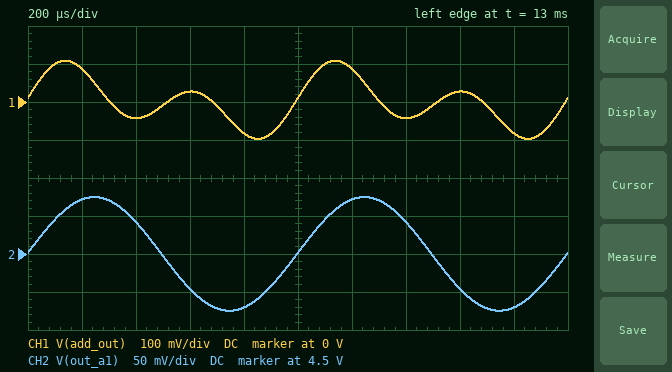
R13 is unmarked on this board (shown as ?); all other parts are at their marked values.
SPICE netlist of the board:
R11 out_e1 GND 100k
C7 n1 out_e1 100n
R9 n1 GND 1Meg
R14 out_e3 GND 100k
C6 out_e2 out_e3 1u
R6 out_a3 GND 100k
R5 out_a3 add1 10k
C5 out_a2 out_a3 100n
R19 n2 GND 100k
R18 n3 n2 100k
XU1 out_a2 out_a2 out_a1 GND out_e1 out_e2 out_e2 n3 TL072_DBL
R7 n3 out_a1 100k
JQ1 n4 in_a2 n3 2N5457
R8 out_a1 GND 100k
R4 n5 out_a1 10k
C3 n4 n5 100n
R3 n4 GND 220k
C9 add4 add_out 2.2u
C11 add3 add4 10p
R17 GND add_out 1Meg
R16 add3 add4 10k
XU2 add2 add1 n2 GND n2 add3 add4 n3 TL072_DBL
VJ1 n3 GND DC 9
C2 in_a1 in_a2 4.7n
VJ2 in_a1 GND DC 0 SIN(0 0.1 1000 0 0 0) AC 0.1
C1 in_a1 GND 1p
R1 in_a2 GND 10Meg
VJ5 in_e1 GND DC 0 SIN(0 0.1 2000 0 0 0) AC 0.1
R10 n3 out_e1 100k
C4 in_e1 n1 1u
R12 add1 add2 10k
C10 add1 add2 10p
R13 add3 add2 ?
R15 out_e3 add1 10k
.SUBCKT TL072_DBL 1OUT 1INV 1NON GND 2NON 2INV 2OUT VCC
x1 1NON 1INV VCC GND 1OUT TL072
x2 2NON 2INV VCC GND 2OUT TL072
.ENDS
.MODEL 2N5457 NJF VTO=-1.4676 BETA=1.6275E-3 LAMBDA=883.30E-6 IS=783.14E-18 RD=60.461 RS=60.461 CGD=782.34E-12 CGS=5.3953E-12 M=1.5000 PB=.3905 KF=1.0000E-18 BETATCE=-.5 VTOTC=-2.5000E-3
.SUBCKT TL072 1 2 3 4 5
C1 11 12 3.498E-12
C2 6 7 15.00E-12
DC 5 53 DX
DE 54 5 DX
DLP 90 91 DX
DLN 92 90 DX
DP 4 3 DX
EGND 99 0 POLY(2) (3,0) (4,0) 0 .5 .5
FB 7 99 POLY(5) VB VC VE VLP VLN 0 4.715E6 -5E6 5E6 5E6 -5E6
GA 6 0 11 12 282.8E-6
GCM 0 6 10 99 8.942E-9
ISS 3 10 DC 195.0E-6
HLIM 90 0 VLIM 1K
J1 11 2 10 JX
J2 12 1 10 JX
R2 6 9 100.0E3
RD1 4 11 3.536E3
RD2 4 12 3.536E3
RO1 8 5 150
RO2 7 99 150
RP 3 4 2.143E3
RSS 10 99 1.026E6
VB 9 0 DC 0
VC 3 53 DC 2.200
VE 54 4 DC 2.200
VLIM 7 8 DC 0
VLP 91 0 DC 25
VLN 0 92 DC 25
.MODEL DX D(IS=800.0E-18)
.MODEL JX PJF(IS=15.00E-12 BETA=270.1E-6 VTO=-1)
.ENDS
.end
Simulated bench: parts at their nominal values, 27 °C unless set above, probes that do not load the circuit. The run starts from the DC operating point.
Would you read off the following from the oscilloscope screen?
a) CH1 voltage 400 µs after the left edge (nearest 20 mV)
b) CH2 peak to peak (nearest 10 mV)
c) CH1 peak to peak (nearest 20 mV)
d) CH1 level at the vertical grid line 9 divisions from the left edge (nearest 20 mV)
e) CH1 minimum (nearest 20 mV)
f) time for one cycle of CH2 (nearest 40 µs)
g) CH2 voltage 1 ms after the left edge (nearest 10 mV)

-40 mV
150 mV
200 mV
-80 mV
-100 mV
1.00 ms
4.50 V
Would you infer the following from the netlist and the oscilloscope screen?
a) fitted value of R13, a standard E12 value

15 kΩ
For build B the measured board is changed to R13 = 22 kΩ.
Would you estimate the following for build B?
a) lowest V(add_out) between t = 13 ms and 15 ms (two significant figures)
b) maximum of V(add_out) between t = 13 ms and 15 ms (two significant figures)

-66 mV
74 mV
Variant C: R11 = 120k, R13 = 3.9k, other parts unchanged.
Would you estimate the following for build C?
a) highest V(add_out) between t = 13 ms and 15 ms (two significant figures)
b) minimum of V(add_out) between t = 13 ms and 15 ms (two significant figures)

420 mV
-370 mV
